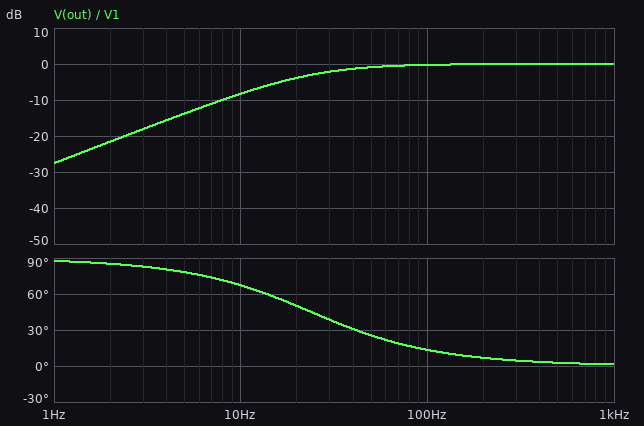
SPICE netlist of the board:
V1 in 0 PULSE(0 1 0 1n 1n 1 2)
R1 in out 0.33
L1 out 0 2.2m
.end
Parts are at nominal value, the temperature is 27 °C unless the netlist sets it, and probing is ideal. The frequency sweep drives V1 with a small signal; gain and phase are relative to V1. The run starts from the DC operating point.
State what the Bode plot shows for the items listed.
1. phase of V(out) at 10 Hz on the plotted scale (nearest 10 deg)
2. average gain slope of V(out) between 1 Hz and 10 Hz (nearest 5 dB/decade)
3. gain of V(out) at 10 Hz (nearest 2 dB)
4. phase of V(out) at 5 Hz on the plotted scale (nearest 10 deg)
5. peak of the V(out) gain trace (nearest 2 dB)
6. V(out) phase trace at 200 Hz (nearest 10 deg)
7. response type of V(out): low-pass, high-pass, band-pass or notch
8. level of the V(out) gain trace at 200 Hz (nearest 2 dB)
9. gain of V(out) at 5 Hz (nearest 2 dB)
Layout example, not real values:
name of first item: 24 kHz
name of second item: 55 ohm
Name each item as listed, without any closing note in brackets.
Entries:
phase of V(out) at 10 Hz on the plotted scale: 70 deg
average gain slope of V(out) between 1 Hz and 10 Hz: 20 dB/decade
gain of V(out) at 10 Hz: -8 dB
phase of V(out) at 5 Hz on the plotted scale: 80 deg
peak of the V(out) gain trace: 0 dB
V(out) phase trace at 200 Hz: 10 deg
response type of V(out): low-pass, high-pass, band-pass or notch: high-pass
level of the V(out) gain trace at 200 Hz: 0 dB
gain of V(out) at 5 Hz: -14 dB
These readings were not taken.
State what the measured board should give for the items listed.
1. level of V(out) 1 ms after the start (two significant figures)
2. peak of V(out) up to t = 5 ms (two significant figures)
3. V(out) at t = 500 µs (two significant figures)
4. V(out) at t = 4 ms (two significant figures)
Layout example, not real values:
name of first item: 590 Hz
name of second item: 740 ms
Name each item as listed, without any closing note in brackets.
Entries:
level of V(out) 1 ms after the start: 860 mV
peak of V(out) up to t = 5 ms: 1.0 V
V(out) at t = 500 µs: 930 mV
V(out) at t = 4 ms: 550 mV
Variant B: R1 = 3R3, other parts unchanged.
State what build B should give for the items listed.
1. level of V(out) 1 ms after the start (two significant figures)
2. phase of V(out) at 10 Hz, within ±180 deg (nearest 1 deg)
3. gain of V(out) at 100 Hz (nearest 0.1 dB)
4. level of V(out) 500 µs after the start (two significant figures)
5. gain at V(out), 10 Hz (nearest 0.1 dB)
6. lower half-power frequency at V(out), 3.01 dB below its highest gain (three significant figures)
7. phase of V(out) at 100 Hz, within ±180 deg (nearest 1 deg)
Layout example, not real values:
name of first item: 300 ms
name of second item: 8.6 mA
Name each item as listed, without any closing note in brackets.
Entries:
level of V(out) 1 ms after the start: 220 mV
phase of V(out) at 10 Hz, within ±180 deg: 88 deg
gain of V(out) at 100 Hz: -8.3 dB
level of V(out) 500 µs after the start: 470 mV
gain at V(out), 10 Hz: -27.6 dB
lower half-power frequency at V(out), 3.01 dB below its highest gain: 239 Hz
phase of V(out) at 100 Hz, within ±180 deg: 67 deg
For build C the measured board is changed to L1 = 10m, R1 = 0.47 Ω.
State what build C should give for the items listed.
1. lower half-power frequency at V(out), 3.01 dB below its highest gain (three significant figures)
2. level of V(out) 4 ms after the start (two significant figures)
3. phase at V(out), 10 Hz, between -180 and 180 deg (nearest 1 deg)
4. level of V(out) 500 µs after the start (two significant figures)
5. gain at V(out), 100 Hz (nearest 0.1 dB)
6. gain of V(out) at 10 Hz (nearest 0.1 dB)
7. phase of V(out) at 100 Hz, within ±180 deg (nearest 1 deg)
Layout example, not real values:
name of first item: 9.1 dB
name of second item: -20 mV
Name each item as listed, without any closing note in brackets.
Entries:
lower half-power frequency at V(out), 3.01 dB below its highest gain: 7.48 Hz
level of V(out) 4 ms after the start: 830 mV
phase at V(out), 10 Hz, between -180 and 180 deg: 37 deg
level of V(out) 500 µs after the start: 980 mV
gain at V(out), 100 Hz: 0 dB
gain of V(out) at 10 Hz: -1.9 dB
phase of V(out) at 100 Hz, within ±180 deg: 4 deg
